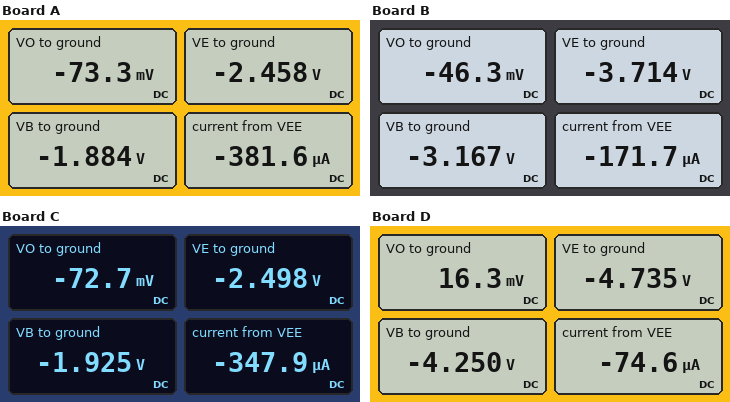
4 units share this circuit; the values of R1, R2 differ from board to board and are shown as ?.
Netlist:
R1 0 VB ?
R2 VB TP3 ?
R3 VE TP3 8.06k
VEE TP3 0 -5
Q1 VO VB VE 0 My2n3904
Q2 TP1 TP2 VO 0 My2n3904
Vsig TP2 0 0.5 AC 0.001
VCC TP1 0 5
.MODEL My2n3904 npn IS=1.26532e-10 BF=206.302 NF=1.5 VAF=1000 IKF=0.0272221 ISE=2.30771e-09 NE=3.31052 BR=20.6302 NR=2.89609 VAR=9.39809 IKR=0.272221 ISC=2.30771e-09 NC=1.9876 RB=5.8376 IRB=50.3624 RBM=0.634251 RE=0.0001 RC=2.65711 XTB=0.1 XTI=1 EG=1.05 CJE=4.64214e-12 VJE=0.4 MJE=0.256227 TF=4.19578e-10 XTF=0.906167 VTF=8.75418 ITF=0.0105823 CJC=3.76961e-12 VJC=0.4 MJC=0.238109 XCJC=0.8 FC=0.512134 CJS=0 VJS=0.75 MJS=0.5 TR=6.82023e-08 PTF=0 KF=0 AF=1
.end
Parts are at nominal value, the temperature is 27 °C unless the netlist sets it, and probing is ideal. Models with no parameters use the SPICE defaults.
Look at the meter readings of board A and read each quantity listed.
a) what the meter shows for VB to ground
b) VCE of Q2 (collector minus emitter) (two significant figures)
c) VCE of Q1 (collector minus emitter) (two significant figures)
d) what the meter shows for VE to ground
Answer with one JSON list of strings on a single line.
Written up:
["-1.884 V", "5.1 V", "2.4 V", "-2.458 V"]
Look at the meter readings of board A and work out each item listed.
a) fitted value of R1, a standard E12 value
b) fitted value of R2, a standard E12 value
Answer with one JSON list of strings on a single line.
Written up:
["27 kΩ", "47 kΩ"]
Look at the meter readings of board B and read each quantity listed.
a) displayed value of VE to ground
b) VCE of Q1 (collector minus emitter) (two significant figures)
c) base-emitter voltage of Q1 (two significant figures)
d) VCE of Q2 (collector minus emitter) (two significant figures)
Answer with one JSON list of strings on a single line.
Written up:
["-3.714 V", "3.7 V", "550 mV", "5.0 V"]
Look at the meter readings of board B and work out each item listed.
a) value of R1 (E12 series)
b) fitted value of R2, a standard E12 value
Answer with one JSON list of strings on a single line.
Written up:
["220 kΩ", "150 kΩ"]
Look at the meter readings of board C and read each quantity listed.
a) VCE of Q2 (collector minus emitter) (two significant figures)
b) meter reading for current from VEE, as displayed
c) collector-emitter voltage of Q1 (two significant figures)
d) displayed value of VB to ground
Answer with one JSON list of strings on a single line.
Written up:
["5.1 V", "-347.9 µA", "2.4 V", "-1.925 V"]
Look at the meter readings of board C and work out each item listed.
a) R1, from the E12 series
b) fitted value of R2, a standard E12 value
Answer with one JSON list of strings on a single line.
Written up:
["47 kΩ", "82 kΩ"]
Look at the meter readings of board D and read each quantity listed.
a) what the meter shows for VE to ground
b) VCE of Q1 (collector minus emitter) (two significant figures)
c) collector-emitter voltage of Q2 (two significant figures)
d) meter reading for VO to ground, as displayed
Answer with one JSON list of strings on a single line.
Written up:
["-4.735 V", "4.8 V", "5.0 V", "16.3 mV"]
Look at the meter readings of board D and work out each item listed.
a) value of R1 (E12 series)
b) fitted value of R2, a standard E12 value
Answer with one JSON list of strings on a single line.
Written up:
["100 kΩ", "18 kΩ"]
